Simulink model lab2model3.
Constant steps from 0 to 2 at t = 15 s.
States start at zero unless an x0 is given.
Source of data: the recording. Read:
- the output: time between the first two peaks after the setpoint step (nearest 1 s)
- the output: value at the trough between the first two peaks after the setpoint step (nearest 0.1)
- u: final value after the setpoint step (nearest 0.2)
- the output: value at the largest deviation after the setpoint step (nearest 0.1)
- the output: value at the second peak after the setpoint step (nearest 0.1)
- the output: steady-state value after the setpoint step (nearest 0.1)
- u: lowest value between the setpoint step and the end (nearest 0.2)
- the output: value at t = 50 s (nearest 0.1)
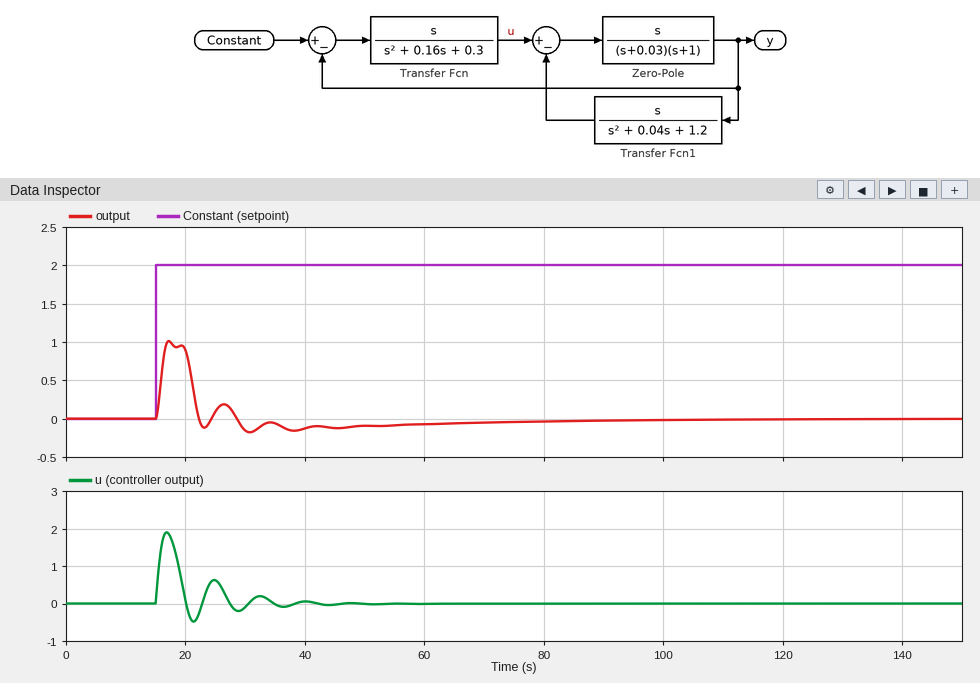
9 s
-0.1
0.0
1.0
0.2
0.0
-0.4
-0.1
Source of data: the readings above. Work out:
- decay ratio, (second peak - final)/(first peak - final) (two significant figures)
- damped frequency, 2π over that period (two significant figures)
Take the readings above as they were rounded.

0.20
0.70 rad/s
